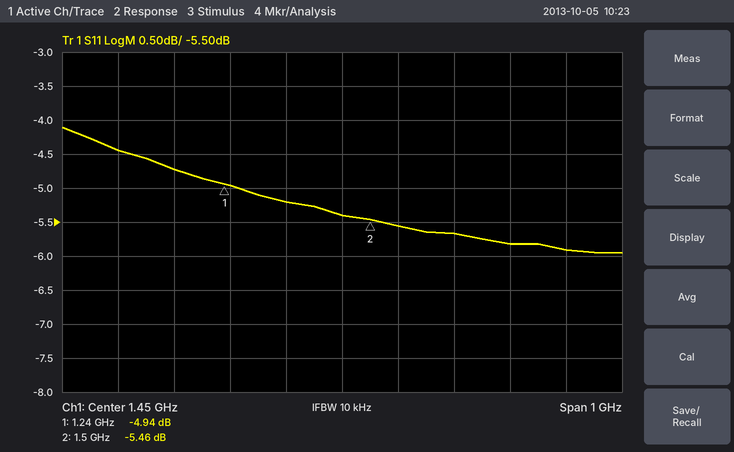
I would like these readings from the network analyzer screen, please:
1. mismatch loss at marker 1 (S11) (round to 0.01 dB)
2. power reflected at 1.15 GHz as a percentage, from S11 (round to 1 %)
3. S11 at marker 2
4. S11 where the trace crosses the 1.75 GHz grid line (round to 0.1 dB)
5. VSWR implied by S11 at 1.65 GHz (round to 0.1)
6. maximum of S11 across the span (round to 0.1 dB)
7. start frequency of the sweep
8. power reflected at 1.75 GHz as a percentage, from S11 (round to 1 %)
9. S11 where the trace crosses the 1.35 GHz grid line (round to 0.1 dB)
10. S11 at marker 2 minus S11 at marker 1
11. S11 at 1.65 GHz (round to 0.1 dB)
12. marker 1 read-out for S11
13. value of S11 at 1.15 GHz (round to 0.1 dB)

1.68 dB
34 %
-5.46 dB
-5.8 dB
3.2
-4.1 dB
950 MHz
26 %
-5.2 dB
-0.52 dB
-5.7 dB
-4.94 dB
-4.7 dB
